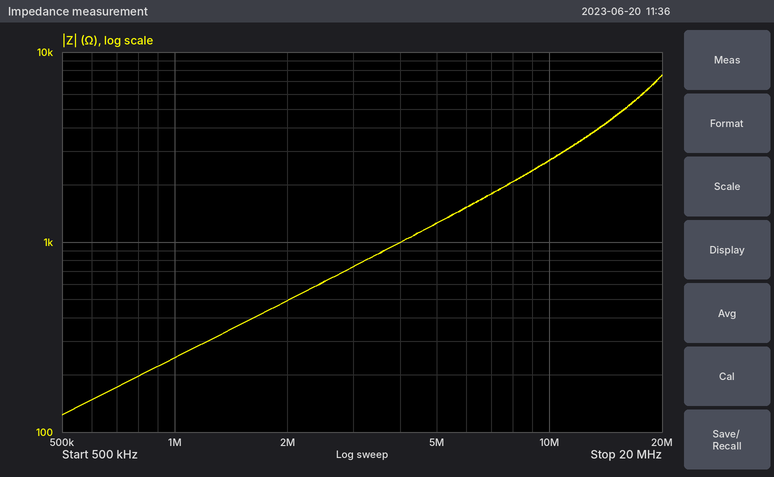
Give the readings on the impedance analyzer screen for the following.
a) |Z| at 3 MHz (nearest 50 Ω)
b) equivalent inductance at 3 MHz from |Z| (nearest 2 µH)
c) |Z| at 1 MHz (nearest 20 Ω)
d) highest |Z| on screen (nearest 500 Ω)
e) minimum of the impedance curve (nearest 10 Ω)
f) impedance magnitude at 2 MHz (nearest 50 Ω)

750 Ω
40 µH
240 Ω
7.5 kΩ
120 Ω
500 Ω
